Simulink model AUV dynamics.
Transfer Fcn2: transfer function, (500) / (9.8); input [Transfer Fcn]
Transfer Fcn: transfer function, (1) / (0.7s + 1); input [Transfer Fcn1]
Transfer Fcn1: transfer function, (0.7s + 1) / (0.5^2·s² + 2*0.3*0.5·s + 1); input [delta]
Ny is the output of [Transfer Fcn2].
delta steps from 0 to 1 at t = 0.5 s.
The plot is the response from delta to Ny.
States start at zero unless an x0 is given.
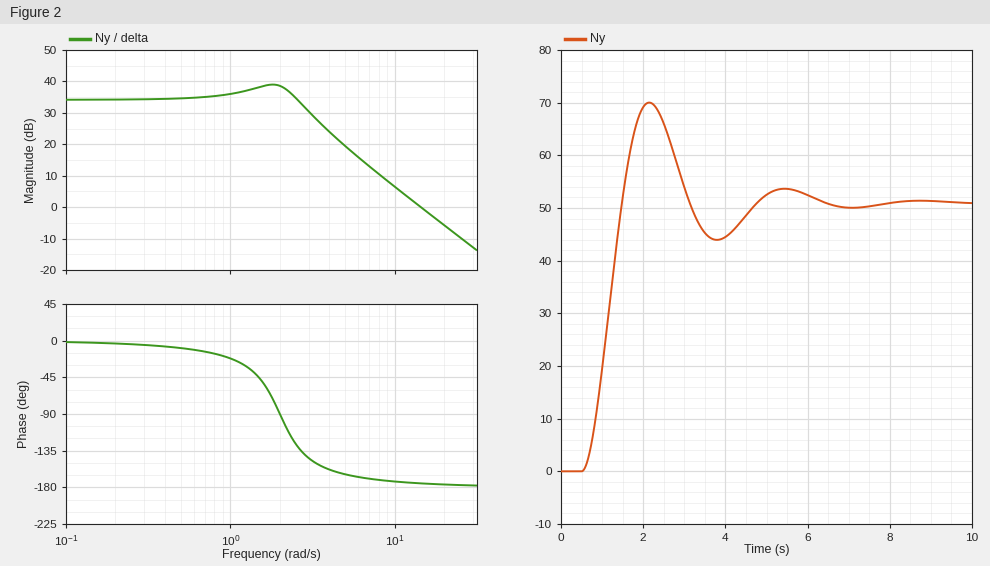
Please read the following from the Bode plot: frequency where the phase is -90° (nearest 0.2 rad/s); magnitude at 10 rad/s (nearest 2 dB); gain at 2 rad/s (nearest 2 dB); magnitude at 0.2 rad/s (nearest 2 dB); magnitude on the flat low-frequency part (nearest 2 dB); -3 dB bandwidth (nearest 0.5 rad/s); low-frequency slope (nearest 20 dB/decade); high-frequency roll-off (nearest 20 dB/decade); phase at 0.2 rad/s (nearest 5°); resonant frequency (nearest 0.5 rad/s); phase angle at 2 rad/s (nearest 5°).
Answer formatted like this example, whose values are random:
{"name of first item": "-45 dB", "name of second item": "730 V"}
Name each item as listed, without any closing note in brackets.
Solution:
{"frequency where the phase is -90°": "2.0 rad/s", "magnitude at 10 rad/s": "6 dB", "gain at 2 rad/s": "38 dB", "magnitude at 0.2 rad/s": "34 dB", "magnitude on the flat low-frequency part": "34 dB", "-3 dB bandwidth": "3.0 rad/s", "low-frequency slope": "0 dB/decade", "high-frequency roll-off": "-40 dB/decade", "phase at 0.2 rad/s": "-5°", "resonant frequency": "2.0 rad/s", "phase angle at 2 rad/s": "-90°"}
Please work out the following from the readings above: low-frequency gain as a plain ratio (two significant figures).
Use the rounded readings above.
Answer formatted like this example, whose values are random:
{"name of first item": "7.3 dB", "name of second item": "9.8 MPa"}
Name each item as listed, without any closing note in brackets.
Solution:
{"low-frequency gain as a plain ratio": "50"}
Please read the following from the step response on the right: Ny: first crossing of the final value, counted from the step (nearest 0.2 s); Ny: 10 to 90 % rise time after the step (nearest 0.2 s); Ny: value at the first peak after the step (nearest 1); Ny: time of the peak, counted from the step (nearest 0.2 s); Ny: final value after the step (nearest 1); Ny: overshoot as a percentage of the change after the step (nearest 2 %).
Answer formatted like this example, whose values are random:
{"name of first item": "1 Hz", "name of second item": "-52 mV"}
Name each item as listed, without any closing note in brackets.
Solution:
{"Ny: first crossing of the final value, counted from the step": "1.0 s", "Ny: 10 to 90 % rise time after the step": "0.6 s", "Ny: value at the first peak after the step": "70", "Ny: time of the peak, counted from the step": "1.6 s", "Ny: final value after the step": "51", "Ny: overshoot as a percentage of the change after the step": "38 %"}
